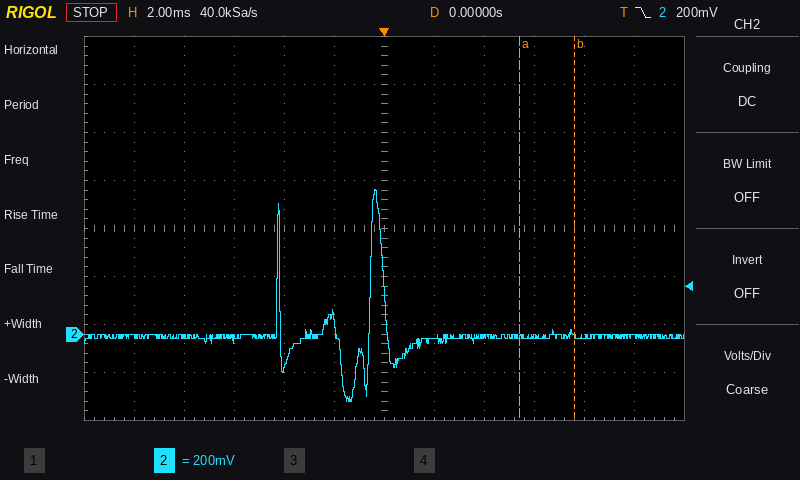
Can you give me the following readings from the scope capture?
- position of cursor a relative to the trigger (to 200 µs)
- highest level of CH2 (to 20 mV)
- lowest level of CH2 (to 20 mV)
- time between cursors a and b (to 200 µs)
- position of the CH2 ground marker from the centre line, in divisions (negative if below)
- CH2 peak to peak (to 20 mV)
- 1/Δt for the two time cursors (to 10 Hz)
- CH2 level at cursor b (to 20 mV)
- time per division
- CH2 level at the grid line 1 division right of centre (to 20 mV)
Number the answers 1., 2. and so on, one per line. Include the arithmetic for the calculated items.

1. +5.4 ms
2. 600 mV
3. -280 mV
4. 2.2 ms
5. -2.2 div
6. 600 mV − (-280 mV) = 880 mV
7. 1 / 2.2 ms ≈ 450 Hz
8. 0 mV
9. 2 ms
10. -20 mV
